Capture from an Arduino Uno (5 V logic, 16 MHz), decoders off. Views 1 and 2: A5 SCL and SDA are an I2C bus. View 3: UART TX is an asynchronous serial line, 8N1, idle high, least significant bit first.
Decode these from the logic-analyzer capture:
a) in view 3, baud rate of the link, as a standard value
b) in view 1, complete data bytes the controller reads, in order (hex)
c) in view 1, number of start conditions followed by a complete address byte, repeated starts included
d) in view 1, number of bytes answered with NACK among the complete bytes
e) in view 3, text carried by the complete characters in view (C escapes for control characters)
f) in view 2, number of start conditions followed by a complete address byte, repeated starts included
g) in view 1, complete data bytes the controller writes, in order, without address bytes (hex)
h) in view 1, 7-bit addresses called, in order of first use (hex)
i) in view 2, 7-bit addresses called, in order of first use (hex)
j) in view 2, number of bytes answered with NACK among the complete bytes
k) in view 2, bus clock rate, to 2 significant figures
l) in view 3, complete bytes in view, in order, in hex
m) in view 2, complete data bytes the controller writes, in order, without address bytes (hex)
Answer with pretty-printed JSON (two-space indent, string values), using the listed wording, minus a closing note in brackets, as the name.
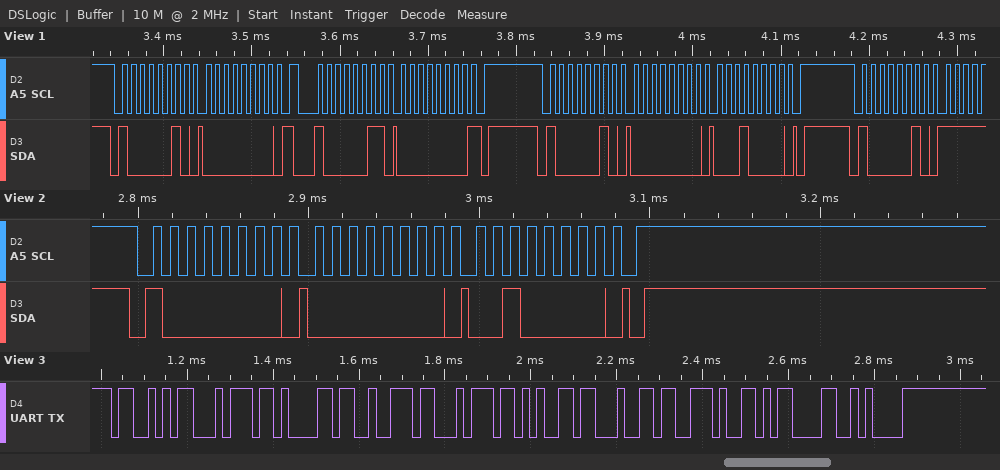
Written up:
{
  "in view 3, baud rate of the link, as a standard value": "57600 baud",
  "in view 1, complete data bytes the controller reads, in order": "00",
  "in view 1, number of start conditions followed by a complete address byte, repeated starts included": "4",
  "in view 1, number of bytes answered with NACK among the complete bytes": "1",
  "in view 3, text carried by the complete characters in view": "\"Started.\\r\\n\"",
  "in view 2, number of start conditions followed by a complete address byte, repeated starts included": "1",
  "in view 1, complete data bytes the controller writes, in order, without address bytes": "00 00 10",
  "in view 1, 7-bit addresses called, in order of first use": "0x41",
  "in view 2, 7-bit addresses called, in order of first use": "0x40",
  "in view 2, number of bytes answered with NACK among the complete bytes": "0",
  "in view 2, bus clock rate, to 2 significant figures": "100 kHz",
  "in view 3, complete bytes in view, in order, in hex": "0x53 0x74 0x61 0x72 0x74 0x65 0x64 0x2E 0x0D 0x0A",
  "in view 2, complete data bytes the controller writes, in order, without address bytes": "00 20"
}
